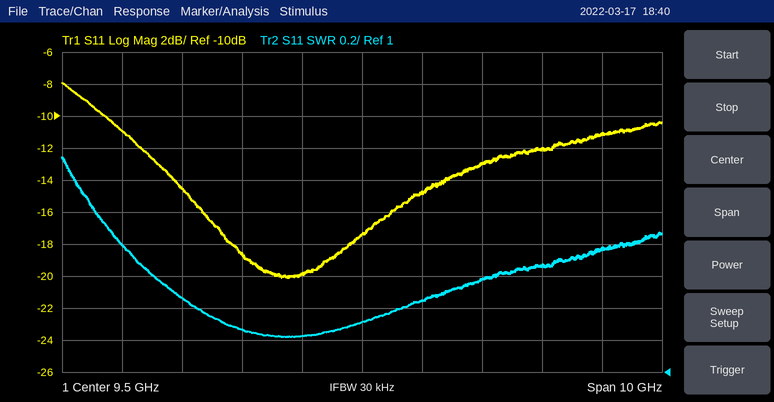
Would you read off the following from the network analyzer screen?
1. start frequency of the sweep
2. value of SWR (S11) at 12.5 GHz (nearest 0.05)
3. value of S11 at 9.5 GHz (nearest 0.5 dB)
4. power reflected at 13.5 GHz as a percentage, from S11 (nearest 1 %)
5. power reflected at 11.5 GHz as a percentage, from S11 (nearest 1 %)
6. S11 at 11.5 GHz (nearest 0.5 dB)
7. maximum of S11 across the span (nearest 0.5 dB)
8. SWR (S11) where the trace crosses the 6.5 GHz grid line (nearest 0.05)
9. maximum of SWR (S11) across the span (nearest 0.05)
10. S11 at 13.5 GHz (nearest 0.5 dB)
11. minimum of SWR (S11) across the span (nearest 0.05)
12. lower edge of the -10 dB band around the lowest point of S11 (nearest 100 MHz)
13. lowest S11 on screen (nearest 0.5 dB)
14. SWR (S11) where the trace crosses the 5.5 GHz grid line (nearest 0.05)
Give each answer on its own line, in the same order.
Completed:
4.5 GHz
1.65
-17.5 dB
8 %
5 %
-13.0 dB
-8.0 dB
1.45
2.35
-11.0 dB
1.20
5.2 GHz
-20.0 dB
1.80
